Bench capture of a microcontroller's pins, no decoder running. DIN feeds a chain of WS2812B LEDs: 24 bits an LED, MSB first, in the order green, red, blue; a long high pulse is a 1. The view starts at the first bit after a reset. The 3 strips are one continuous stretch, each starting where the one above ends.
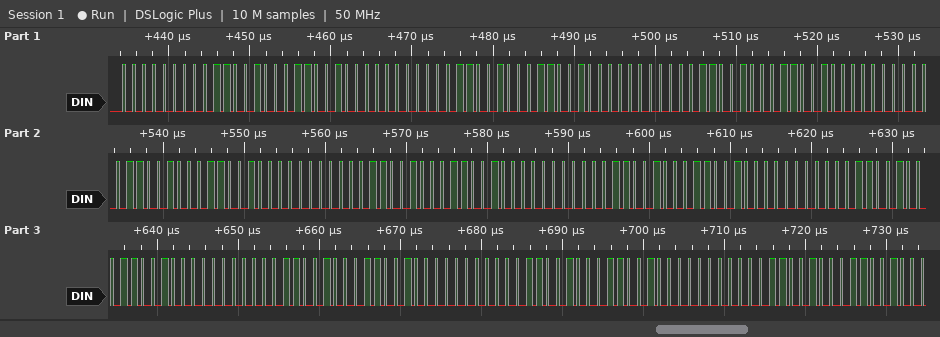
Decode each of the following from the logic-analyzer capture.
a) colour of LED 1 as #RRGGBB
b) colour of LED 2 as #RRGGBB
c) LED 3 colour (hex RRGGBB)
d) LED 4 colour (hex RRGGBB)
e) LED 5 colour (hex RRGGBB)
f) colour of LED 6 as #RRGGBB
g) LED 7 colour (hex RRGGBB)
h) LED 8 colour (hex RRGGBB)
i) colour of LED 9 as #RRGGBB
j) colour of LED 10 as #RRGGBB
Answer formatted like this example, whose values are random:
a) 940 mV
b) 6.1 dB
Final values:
a) #640064
b) #640064
c) #640064
d) #640064
e) #640064
f) #640064
g) #640064
h) #640064
i) #640064
j) #640064
